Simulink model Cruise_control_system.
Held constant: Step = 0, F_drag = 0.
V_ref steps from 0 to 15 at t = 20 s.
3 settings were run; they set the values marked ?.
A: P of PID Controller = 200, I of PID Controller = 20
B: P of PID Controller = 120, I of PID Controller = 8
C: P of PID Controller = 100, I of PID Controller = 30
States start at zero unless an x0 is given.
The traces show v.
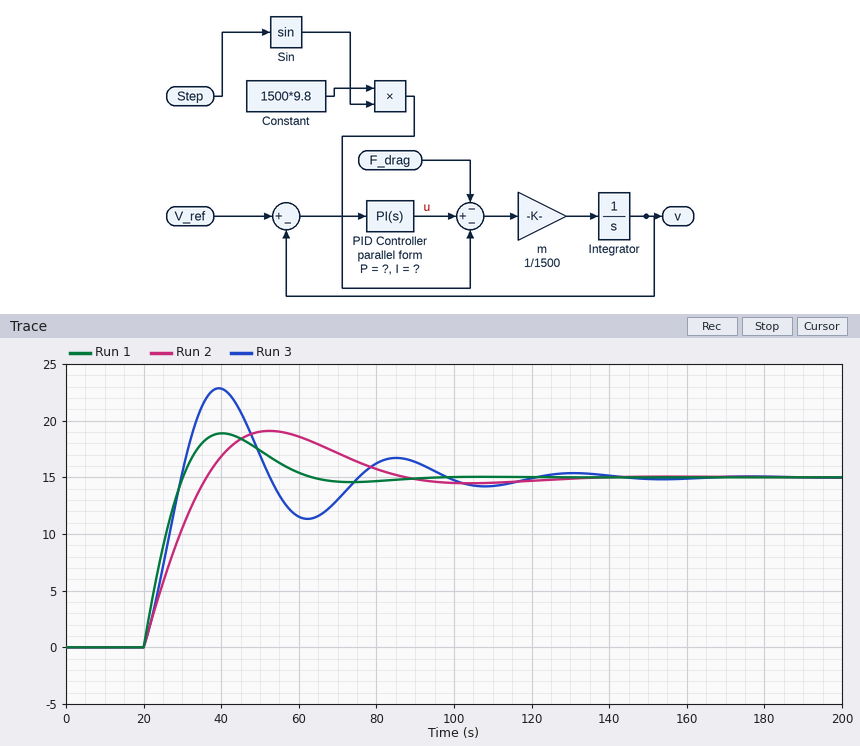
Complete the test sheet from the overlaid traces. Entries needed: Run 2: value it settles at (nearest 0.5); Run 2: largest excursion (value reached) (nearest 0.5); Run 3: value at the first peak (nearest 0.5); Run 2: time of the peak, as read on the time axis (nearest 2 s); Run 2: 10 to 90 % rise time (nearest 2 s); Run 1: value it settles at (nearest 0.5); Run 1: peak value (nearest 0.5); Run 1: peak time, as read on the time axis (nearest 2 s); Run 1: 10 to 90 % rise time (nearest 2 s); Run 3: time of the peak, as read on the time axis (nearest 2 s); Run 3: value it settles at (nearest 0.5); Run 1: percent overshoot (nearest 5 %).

15.0
19.0
23.0
52 s
12 s
15.0
19.0
40 s
8 s
40 s
15.0
25 %
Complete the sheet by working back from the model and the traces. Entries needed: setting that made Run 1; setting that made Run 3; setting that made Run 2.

A
C
B
